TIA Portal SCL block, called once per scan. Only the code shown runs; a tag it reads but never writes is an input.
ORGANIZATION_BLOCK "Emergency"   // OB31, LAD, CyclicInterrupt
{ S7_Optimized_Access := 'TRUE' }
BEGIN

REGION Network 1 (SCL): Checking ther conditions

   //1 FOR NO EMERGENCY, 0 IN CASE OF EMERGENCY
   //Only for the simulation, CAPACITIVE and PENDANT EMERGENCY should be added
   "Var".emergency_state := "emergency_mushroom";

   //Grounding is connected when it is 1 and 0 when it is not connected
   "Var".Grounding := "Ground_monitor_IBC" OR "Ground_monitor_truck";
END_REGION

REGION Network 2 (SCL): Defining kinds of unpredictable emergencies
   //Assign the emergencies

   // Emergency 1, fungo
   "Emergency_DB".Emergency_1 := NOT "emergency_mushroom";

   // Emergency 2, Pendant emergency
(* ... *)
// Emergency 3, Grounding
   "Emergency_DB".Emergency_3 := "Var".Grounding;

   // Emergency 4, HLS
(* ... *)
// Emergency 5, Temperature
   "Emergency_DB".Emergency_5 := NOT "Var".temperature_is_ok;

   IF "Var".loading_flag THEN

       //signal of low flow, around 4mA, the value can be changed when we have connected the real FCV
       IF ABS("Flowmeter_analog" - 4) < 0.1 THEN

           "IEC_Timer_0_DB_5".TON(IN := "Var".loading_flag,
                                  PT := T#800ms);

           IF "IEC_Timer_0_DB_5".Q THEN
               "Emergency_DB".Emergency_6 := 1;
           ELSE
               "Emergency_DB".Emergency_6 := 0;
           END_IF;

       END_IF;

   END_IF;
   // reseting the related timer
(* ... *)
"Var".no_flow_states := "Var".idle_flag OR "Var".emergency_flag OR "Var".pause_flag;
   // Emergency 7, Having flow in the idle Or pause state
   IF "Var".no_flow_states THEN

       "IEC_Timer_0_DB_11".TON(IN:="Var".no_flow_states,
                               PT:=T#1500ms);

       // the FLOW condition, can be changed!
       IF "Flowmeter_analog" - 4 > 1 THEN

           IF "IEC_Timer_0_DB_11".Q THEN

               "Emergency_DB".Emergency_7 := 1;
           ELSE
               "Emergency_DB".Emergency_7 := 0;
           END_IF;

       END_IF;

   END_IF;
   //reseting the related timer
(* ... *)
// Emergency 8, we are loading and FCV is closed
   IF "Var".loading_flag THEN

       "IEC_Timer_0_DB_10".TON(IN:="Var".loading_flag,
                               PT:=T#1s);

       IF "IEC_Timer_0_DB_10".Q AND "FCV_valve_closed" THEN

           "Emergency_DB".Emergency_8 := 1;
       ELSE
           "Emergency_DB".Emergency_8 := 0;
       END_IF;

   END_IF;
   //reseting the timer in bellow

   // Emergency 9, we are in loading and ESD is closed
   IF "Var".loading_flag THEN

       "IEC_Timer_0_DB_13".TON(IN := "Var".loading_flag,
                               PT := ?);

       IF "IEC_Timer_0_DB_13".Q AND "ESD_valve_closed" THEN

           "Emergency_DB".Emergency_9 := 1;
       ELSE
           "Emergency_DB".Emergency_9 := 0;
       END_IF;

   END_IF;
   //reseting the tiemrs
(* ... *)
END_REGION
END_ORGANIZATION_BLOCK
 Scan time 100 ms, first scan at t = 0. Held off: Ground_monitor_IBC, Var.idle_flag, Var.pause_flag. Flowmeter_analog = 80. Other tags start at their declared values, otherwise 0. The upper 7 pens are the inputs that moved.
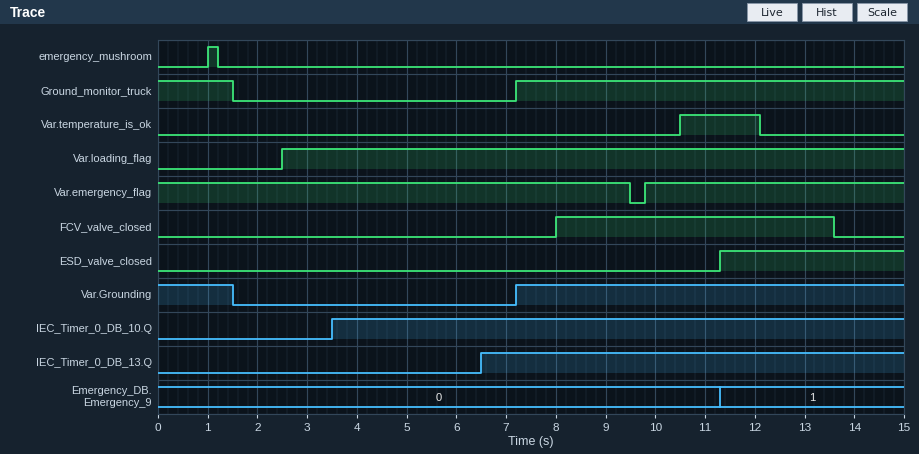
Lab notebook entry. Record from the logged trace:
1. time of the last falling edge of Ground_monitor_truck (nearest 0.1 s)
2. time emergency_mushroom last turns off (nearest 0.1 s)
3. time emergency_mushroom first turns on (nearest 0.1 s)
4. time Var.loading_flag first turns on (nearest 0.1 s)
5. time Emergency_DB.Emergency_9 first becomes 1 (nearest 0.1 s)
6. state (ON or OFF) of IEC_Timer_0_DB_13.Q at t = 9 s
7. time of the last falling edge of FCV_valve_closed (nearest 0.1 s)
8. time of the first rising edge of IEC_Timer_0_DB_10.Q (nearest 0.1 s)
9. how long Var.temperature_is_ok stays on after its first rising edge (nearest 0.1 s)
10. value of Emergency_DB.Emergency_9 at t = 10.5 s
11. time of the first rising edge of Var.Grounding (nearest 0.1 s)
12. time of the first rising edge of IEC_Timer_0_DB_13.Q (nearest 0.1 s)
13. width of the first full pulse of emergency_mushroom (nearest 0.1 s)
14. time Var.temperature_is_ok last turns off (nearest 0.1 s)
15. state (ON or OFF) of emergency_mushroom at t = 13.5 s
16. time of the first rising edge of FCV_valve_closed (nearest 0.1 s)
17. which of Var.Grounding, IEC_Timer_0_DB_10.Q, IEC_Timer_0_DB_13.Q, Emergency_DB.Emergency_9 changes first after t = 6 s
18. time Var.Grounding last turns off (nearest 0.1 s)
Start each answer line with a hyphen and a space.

- 1.5 s
- 1.2 s
- 1.0 s
- 2.5 s
- 11.3 s
- ON
- 13.6 s
- 3.5 s
- 1.6 s
- 0
- 7.2 s
- 6.5 s
- 0.2 s
- 12.1 s
- OFF
- 8.0 s
- IEC_Timer_0_DB_13.Q
- 1.5 s
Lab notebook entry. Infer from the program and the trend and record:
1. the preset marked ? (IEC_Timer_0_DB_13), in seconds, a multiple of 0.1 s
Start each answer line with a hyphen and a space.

- 4.0 s
